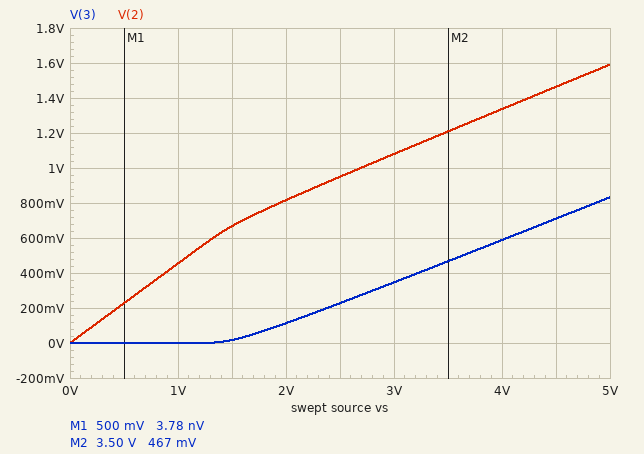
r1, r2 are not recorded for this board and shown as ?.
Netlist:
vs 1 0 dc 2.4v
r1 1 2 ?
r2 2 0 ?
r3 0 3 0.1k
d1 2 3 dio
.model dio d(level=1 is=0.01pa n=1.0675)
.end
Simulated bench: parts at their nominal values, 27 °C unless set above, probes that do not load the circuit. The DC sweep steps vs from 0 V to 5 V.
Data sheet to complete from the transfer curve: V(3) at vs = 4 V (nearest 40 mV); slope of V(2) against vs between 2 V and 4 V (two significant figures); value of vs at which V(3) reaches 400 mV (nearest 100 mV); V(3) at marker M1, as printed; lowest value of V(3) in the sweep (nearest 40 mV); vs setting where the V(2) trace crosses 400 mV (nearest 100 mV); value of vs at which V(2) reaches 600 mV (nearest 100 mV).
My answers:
600 mV
0.26 V/V
3.2 V
3.78 nV
0 V
900 mV
1.3 V
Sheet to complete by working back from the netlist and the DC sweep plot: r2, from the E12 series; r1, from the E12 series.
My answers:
150 Ω
180 Ω
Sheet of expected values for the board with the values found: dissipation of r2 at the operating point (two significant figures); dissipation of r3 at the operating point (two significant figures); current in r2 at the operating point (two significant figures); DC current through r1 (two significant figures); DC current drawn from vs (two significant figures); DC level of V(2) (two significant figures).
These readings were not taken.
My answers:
5.7 mW
420 µW
6.2 mA
8.2 mA
8.2 mA
920 mV
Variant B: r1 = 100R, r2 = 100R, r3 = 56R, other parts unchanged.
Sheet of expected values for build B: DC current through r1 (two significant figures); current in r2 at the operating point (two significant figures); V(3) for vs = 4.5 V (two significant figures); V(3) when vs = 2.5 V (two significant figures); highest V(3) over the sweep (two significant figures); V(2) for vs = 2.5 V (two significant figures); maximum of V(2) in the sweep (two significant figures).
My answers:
14 mA
9.8 mA
780 mV
270 mV
910 mV
1.0 V
1.7 V
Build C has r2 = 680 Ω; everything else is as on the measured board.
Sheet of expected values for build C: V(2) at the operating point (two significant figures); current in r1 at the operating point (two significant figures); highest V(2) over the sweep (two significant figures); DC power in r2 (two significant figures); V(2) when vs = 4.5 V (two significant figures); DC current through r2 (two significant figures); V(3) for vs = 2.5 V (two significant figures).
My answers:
1.2 V
6.6 mA
2.1 V
2.2 mW
1.9 V
1.8 mA
510 mV
